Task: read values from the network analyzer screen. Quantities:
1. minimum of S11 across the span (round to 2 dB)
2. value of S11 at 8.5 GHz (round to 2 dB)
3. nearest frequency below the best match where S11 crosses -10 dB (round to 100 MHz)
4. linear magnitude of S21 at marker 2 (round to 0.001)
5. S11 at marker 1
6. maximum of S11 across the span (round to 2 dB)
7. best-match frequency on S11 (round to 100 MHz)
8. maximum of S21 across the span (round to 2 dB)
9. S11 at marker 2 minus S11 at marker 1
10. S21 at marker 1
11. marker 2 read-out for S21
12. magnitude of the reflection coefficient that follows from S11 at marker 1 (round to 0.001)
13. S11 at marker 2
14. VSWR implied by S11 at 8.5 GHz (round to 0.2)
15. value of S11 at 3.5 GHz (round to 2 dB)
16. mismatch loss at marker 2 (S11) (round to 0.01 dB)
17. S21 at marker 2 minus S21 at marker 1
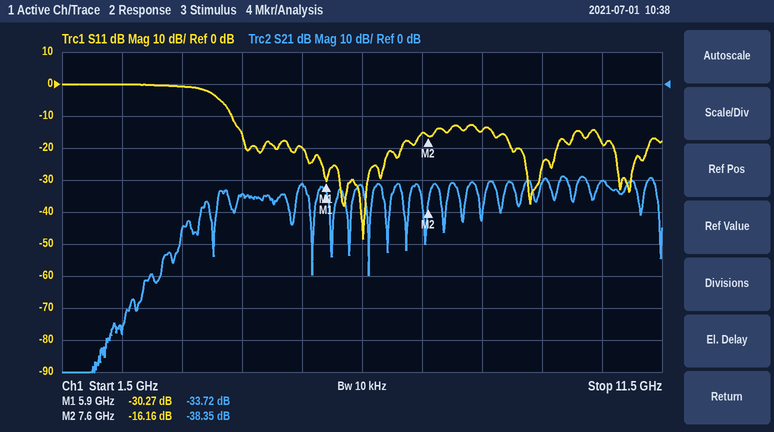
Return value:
-48 dB
-14 dB
4.3 GHz
0.012
-30.27 dB
0 dB
6.5 GHz
-28 dB
14.11 dB
-33.72 dB
-38.35 dB
0.031
-16.16 dB
1.4
0 dB
0.11 dB
-4.63 dB
